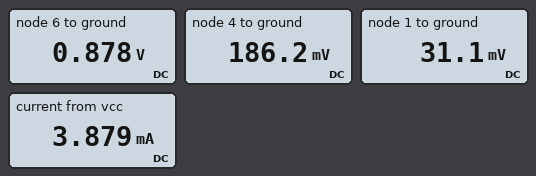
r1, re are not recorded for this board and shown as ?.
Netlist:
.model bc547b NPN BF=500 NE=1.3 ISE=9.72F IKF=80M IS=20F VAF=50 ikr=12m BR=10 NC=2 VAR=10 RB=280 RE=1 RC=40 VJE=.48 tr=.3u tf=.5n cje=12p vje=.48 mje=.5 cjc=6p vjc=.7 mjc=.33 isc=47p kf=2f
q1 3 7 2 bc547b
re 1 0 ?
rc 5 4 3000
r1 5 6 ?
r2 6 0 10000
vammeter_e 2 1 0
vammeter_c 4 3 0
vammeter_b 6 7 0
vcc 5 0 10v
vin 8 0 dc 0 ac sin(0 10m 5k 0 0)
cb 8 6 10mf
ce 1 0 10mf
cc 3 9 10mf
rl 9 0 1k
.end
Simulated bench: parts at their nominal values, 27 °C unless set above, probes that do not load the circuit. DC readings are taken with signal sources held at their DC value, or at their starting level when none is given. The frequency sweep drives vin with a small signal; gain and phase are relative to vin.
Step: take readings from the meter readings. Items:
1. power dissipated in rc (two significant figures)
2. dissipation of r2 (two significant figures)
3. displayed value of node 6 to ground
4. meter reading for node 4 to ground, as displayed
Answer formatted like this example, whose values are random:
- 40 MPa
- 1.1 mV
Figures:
- 32 mW
- 77 µW
- 0.878 V
- 186.2 mV
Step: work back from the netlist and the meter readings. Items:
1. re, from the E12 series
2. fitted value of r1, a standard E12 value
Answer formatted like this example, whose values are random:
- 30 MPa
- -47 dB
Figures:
- 8.2 Ω
- 15 kΩ
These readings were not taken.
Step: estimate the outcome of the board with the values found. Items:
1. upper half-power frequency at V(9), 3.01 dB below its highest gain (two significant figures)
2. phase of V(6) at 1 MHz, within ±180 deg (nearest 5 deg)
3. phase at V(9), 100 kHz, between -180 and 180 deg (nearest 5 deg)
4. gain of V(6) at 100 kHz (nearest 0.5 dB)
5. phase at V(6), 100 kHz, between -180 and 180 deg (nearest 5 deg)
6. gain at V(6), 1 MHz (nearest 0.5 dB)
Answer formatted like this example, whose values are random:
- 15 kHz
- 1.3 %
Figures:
- 68 kHz
- 0 deg
- 95 deg
- 0 dB
- 0 deg
- 0 dB
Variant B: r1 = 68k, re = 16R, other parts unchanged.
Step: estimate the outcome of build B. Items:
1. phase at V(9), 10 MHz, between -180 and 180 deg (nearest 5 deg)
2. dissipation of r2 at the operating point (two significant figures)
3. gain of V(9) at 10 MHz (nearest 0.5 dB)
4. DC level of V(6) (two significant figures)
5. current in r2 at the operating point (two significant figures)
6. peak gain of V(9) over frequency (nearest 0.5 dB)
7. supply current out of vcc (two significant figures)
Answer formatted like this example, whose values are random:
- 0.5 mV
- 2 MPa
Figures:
- 15 deg
- 56 µW
- -31.0 dB
- 750 mV
- 75 µA
- 2.0 dB
- 3.4 mA
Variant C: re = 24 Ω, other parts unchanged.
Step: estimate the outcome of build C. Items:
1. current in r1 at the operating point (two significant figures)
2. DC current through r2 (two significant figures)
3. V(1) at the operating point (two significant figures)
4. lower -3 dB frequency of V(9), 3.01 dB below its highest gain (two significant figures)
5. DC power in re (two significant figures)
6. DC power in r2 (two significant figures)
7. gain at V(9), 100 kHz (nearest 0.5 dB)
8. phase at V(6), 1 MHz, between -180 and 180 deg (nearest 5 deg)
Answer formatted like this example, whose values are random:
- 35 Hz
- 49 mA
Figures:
- 600 µA
- 93 µA
- 90 mV
- 700 mHz
- 340 µW
- 87 µW
- -29.5 dB
- 0 deg
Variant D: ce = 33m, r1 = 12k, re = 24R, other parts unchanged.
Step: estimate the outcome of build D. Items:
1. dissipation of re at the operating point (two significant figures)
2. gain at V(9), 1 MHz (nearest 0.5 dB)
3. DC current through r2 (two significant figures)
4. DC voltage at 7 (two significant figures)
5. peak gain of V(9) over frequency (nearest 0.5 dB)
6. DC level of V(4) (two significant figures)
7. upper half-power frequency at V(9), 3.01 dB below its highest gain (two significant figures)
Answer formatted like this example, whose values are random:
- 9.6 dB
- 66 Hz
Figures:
- 370 µW
- -36.5 dB
- 98 µA
- 980 mV
- -28.5 dB
- 250 mV
- 74 kHz
